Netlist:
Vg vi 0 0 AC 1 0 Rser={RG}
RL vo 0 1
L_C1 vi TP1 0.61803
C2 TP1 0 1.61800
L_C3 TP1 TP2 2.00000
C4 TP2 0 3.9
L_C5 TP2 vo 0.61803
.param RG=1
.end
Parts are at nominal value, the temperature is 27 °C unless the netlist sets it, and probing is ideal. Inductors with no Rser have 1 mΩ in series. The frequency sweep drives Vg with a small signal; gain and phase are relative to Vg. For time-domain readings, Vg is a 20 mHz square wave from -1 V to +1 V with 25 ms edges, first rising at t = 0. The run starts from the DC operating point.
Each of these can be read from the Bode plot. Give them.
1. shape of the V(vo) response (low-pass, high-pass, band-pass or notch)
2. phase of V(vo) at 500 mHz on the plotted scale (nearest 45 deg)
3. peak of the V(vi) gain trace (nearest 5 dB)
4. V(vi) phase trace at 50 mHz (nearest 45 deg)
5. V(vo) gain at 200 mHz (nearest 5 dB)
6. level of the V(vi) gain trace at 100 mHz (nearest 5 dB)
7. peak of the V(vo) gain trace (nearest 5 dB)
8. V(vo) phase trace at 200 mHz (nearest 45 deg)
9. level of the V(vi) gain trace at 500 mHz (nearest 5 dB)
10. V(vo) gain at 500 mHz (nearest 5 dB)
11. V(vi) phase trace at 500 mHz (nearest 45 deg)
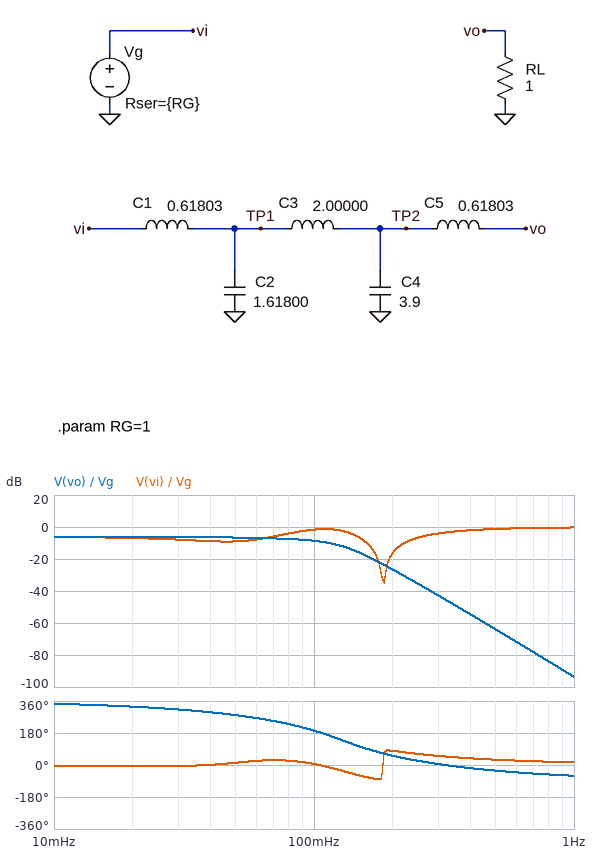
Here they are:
low-pass
-45 deg
0 dB
0 deg
-25 dB
0 dB
-5 dB
45 deg
0 dB
-65 dB
45 deg
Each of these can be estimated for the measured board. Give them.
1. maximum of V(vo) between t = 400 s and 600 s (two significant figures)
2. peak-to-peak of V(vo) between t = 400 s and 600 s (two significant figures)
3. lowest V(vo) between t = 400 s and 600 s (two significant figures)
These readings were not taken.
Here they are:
550 mV
1.1 V
-550 mV
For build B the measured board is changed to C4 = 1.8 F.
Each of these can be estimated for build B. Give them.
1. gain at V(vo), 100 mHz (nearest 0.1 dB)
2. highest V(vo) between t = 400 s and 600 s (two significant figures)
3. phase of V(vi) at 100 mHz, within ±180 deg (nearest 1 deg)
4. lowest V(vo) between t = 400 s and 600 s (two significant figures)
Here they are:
-6.1 dB
630 mV
0 deg
-630 mV
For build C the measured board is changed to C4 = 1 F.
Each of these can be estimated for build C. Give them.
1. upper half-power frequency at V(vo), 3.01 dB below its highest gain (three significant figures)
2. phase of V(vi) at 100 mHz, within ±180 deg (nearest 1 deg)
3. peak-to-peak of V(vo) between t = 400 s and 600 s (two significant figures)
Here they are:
175 mHz
-14 deg
1.2 V
